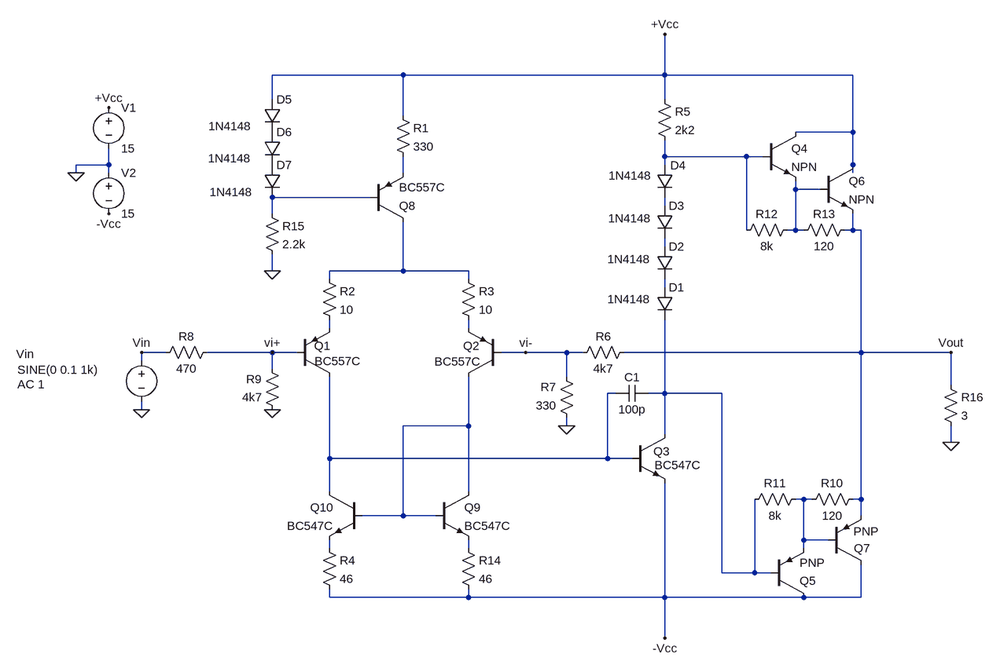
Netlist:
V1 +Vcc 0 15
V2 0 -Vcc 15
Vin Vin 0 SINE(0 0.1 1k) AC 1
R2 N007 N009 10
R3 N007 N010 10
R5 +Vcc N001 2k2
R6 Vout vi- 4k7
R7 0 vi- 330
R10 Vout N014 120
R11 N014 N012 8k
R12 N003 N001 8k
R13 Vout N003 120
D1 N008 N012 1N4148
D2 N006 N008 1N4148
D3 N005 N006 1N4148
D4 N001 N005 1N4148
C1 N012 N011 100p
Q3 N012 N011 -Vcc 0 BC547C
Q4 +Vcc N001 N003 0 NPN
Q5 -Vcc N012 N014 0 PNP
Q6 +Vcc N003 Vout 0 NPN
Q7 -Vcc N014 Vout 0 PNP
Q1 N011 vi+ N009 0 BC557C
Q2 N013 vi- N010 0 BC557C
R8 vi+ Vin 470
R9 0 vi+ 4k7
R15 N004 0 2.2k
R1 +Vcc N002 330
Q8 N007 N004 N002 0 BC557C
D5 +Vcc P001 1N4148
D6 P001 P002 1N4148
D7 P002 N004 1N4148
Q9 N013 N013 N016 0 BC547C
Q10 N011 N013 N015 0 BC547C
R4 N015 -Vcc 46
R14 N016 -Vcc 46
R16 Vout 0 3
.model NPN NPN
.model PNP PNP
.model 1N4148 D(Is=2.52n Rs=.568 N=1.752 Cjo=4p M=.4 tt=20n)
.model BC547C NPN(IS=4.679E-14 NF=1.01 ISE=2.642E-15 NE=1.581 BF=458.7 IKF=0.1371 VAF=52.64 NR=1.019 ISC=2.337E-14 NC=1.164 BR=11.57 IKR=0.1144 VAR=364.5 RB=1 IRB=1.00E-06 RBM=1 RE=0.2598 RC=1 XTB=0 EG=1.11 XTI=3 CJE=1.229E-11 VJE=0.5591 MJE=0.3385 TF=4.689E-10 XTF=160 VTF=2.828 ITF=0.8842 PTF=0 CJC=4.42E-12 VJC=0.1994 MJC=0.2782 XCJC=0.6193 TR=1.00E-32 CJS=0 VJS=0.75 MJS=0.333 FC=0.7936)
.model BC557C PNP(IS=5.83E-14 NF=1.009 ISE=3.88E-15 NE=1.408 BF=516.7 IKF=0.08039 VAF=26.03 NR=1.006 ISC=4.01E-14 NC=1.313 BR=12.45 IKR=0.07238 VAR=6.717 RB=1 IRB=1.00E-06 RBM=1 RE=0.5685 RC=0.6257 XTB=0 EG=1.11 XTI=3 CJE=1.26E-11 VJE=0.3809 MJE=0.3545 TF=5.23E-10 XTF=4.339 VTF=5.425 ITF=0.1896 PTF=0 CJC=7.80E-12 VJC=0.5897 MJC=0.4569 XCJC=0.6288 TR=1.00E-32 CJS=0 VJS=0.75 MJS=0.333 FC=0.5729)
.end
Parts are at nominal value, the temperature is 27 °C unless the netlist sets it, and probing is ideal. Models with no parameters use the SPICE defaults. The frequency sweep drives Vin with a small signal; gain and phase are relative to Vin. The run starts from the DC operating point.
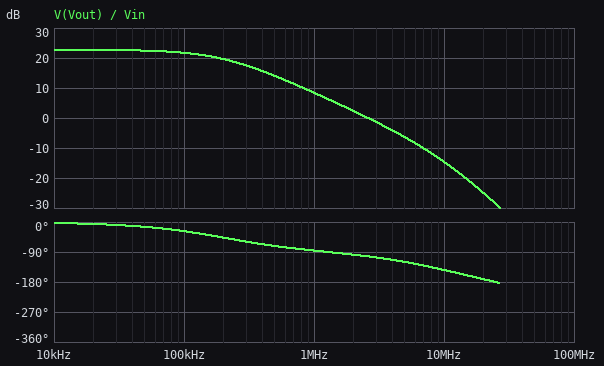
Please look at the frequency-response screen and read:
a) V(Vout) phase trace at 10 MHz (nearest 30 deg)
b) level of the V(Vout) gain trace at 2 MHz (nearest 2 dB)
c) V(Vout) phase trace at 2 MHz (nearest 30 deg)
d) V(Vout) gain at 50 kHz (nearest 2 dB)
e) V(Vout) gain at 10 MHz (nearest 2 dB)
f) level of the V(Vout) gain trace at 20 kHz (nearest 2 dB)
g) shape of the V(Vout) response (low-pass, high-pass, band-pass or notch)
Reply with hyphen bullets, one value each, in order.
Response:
- -150 deg
- 2 dB
- -90 deg
- 22 dB
- -14 dB
- 22 dB
- low-pass
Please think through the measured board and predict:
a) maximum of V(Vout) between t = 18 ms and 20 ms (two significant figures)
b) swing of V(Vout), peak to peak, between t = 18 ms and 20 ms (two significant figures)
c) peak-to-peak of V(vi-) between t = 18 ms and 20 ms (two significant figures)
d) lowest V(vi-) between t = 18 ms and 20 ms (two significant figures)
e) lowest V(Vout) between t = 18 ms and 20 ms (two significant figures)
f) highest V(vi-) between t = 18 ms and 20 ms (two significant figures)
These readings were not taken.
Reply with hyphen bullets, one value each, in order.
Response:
- 1.4 V
- 2.8 V
- 180 mV
- -90 mV
- -1.4 V
- 92 mV
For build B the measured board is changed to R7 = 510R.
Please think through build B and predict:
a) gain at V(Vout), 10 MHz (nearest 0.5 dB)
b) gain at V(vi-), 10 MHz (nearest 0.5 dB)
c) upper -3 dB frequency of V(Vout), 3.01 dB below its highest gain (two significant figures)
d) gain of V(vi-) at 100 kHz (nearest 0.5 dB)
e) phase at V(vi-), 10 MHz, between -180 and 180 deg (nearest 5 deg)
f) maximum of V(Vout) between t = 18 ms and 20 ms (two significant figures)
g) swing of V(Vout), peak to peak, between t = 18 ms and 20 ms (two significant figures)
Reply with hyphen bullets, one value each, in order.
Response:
- -15.5 dB
- -9.0 dB
- 300 kHz
- -1.5 dB
- 35 deg
- 930 mV
- 1.9 V
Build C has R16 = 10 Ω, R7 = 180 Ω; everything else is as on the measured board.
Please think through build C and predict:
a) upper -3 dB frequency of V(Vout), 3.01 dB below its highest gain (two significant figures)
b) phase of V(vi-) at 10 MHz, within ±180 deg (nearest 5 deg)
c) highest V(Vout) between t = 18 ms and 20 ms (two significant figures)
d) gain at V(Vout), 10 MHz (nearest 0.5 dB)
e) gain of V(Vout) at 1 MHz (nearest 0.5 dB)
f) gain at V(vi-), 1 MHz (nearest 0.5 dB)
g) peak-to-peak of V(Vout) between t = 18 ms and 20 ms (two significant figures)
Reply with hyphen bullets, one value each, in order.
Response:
- 340 kHz
- 50 deg
- 2.5 V
- -4.0 dB
- 18.0 dB
- -11.5 dB
- 4.9 V
